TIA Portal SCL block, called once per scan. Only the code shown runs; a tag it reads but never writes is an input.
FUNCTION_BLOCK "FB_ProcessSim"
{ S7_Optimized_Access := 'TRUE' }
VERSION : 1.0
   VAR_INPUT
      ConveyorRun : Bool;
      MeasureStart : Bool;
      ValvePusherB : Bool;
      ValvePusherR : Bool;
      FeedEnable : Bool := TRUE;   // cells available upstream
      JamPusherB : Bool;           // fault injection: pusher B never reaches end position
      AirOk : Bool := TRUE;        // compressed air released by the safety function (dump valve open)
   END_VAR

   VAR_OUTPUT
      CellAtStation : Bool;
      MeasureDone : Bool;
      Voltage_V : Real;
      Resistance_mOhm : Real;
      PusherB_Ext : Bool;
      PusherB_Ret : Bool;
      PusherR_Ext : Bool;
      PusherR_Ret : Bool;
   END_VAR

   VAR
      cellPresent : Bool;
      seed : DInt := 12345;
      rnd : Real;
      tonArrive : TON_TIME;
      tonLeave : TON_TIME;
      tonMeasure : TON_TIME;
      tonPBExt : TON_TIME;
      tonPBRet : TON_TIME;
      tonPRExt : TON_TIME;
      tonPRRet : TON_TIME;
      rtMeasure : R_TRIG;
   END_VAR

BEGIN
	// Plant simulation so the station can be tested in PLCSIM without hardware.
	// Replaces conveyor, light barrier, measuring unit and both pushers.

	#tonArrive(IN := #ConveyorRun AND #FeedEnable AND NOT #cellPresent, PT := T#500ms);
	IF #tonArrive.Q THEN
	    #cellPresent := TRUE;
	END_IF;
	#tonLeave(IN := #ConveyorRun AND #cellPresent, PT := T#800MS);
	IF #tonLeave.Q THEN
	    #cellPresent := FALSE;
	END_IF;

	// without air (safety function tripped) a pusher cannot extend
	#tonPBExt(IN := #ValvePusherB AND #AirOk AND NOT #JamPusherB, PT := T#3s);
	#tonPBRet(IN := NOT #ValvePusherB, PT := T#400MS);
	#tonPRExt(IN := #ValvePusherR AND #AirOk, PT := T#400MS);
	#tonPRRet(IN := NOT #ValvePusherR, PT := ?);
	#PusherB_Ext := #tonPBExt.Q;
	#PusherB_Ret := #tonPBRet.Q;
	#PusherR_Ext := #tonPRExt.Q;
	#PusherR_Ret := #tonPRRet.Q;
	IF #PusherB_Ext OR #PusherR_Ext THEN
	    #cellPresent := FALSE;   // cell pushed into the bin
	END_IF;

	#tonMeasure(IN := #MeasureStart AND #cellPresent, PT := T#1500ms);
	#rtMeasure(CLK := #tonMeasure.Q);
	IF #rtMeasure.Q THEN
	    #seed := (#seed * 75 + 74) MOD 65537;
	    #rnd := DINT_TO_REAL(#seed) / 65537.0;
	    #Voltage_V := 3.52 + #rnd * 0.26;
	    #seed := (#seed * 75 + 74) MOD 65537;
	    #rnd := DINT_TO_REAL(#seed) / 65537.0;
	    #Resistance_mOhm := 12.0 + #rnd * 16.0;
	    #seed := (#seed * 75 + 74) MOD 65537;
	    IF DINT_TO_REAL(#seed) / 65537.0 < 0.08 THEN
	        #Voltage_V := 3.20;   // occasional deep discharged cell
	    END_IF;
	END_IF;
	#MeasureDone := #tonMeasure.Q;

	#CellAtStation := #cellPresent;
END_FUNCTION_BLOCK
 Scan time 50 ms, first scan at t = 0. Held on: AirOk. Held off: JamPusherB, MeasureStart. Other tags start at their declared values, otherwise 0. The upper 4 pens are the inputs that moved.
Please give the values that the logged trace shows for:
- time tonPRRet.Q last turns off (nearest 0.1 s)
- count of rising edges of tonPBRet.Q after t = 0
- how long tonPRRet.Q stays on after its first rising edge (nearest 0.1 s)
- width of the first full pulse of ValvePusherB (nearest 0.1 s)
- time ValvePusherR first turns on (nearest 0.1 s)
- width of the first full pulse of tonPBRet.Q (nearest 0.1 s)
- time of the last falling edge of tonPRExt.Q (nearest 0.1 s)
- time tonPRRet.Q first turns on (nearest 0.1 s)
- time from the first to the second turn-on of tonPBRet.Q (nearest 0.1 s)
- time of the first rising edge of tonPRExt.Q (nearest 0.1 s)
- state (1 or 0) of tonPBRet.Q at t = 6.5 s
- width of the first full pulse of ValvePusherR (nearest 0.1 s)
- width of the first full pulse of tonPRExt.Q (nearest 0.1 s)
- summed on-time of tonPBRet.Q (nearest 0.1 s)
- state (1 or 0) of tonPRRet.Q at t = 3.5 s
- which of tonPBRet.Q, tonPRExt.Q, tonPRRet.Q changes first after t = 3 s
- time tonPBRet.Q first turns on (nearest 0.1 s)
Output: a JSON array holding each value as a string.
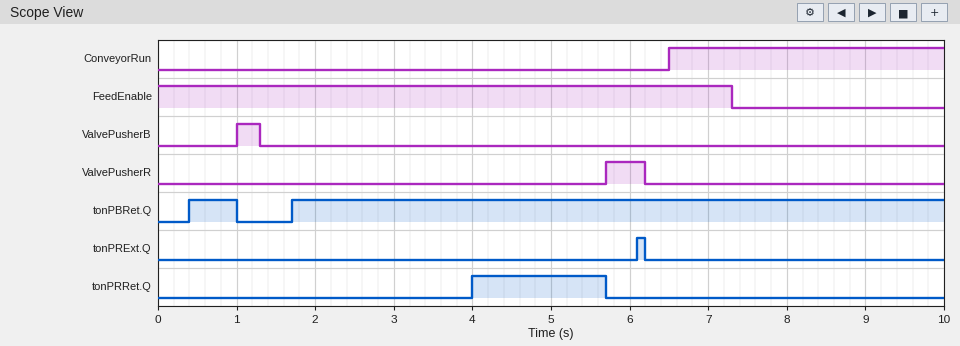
["5.7 s", "2", "1.7 s", "0.3 s", "5.7 s", "0.6 s", "6.2 s", "4.0 s", "1.3 s", "6.1 s", "1", "0.5 s", "0.1 s", "8.9 s", "0", "tonPRRet.Q", "0.4 s"]
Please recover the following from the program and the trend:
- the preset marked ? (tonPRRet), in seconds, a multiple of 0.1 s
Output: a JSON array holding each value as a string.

["4.0 s"]
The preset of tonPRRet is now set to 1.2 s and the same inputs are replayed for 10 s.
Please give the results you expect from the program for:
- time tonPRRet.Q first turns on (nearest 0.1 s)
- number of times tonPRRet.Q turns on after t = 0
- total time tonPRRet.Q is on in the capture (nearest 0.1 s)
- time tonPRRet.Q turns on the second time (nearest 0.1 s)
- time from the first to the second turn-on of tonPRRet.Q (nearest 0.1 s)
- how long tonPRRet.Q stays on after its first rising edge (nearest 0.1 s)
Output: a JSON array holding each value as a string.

["1.2 s", "2", "7.1 s", "7.4 s", "6.2 s", "4.5 s"]
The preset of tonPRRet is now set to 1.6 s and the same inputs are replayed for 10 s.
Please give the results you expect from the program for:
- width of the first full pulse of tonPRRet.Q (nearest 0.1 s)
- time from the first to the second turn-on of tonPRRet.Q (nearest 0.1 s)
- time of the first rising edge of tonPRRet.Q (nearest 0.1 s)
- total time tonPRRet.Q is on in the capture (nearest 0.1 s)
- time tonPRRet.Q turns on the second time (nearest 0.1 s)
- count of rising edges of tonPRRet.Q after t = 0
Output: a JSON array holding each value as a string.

["4.1 s", "6.2 s", "1.6 s", "6.3 s", "7.8 s", "2"]
